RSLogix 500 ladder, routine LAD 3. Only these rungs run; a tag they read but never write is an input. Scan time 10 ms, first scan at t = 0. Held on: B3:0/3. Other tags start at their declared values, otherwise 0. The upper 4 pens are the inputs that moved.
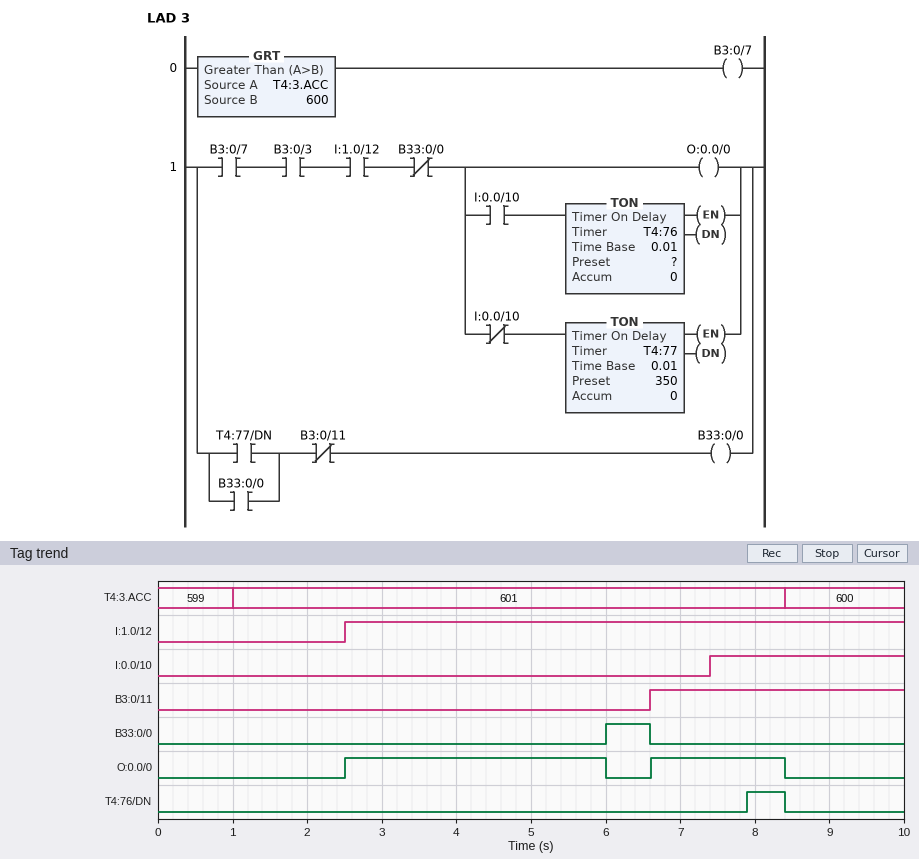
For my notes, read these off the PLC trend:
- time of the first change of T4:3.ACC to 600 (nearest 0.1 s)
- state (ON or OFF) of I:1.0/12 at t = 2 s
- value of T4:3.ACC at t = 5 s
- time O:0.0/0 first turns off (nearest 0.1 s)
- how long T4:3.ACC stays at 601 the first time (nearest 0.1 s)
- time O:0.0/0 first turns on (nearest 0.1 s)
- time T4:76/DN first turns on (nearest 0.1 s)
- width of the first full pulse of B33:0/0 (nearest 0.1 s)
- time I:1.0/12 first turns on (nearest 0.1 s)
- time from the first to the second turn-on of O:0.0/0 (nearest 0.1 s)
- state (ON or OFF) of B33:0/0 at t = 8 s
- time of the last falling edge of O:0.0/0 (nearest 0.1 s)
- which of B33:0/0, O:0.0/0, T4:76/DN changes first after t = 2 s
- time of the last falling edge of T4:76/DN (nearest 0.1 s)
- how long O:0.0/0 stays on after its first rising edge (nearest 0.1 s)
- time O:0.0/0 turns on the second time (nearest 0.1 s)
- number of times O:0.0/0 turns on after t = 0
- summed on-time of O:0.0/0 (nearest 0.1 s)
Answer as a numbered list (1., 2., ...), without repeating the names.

1. 8.4 s
2. OFF
3. 601
4. 6.0 s
5. 7.4 s
6. 2.5 s
7. 7.9 s
8. 0.6 s
9. 2.5 s
10. 4.1 s
11. OFF
12. 8.4 s
13. O:0.0/0
14. 8.4 s
15. 3.5 s
16. 6.6 s
17. 2
18. 5.3 s
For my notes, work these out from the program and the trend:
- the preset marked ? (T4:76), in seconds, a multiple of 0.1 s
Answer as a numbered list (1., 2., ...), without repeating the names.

1. 0.5 s
